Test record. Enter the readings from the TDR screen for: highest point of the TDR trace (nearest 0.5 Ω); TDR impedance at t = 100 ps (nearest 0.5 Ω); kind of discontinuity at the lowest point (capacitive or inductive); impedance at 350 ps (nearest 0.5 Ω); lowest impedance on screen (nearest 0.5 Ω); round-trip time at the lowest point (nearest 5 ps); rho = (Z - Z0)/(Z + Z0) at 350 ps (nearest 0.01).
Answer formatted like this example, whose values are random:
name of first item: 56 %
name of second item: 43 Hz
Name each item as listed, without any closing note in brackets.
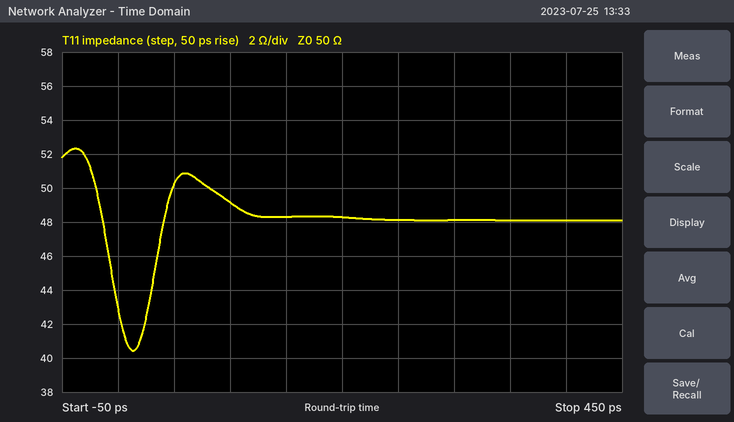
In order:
highest point of the TDR trace: 52.5 Ω
TDR impedance at t = 100 ps: 49.0 Ω
kind of discontinuity at the lowest point: capacitive
impedance at 350 ps: 48.0 Ω
lowest impedance on screen: 40.5 Ω
round-trip time at the lowest point: 15 ps
rho = (Z - Z0)/(Z + Z0) at 350 ps: -0.02
